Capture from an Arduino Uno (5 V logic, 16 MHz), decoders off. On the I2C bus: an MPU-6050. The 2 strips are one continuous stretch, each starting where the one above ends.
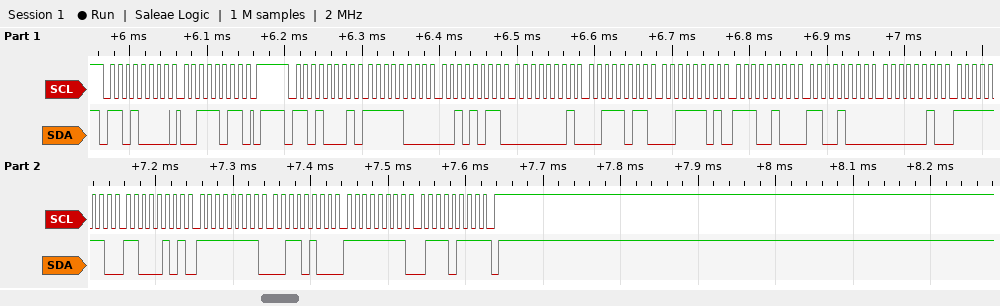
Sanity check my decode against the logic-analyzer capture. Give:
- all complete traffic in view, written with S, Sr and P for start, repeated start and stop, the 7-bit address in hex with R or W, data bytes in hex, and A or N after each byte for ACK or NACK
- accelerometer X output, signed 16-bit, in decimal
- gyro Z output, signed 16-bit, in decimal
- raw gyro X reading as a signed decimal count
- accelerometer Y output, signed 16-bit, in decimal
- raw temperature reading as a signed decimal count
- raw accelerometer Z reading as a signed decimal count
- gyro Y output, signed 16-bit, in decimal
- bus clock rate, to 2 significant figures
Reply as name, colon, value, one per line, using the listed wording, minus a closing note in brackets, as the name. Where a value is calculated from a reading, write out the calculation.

all complete traffic in view, written with S, Sr and P for start, repeated start and stop, the 7-bit address in hex with R or W, data bytes in hex, and A or N after each byte for ACK or NACK: S 68W A 3B A P S 68R A F8 A 2B A 01 A 3B A 3D A E4 A C8 A 02 A FE A C5 A FF A 34 A FF A 77 N P
accelerometer X output, signed 16-bit, in decimal: 0xF82B = -2005
gyro Z output, signed 16-bit, in decimal: 0xFF77 = -137
raw gyro X reading as a signed decimal count: 0xFEC5 = -315
accelerometer Y output, signed 16-bit, in decimal: 0x013B = 315
raw temperature reading as a signed decimal count: 0xC802 = -14334
raw accelerometer Z reading as a signed decimal count: 0x3DE4 = 15844
gyro Y output, signed 16-bit, in decimal: 0xFF34 = -204
bus clock rate, to 2 significant figures: 100 kHz
